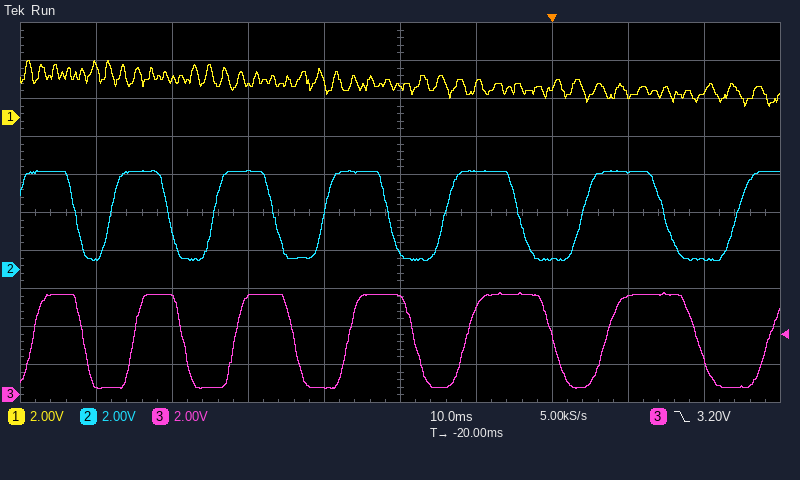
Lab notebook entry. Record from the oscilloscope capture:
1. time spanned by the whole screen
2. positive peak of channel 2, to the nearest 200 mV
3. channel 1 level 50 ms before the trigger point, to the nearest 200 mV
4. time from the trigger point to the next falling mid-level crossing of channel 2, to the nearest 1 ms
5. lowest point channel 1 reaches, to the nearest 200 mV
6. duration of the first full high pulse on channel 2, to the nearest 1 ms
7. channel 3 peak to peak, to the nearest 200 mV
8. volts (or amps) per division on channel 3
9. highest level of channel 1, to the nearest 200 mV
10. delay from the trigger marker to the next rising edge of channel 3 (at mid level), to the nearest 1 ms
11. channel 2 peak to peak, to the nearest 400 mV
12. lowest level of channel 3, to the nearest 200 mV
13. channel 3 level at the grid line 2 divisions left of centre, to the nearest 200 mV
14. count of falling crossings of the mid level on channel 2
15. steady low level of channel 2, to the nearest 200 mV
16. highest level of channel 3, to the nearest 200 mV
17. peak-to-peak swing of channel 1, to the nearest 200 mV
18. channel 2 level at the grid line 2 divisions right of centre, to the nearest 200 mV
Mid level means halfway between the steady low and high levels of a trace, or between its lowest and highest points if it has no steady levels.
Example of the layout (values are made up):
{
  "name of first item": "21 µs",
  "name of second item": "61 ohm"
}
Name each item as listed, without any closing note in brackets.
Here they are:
{
  "time spanned by the whole screen": "100 ms",
  "positive peak of channel 2, to the nearest 200 mV": "5.2 V",
  "channel 1 level 50 ms before the trigger point, to the nearest 200 mV": "2.0 V",
  "time from the trigger point to the next falling mid-level crossing of channel 2, to the nearest 1 ms": "15 ms",
  "lowest point channel 1 reaches, to the nearest 200 mV": "600 mV",
  "duration of the first full high pulse on channel 2, to the nearest 1 ms": "8 ms",
  "channel 3 peak to peak, to the nearest 200 mV": "5.0 V",
  "volts (or amps) per division on channel 3": "2 V",
  "highest level of channel 1, to the nearest 200 mV": "3.0 V",
  "delay from the trigger marker to the next rising edge of channel 3 (at mid level), to the nearest 1 ms": "7 ms",
  "channel 2 peak to peak, to the nearest 400 mV": "4.8 V",
  "lowest level of channel 3, to the nearest 200 mV": "400 mV",
  "channel 3 level at the grid line 2 divisions left of centre, to the nearest 200 mV": "5.2 V",
  "count of falling crossings of the mid level on channel 2": "6",
  "steady low level of channel 2, to the nearest 200 mV": "600 mV",
  "highest level of channel 3, to the nearest 200 mV": "5.4 V",
  "peak-to-peak swing of channel 1, to the nearest 200 mV": "2.4 V",
  "channel 2 level at the grid line 2 divisions right of centre, to the nearest 200 mV": "600 mV"
}
